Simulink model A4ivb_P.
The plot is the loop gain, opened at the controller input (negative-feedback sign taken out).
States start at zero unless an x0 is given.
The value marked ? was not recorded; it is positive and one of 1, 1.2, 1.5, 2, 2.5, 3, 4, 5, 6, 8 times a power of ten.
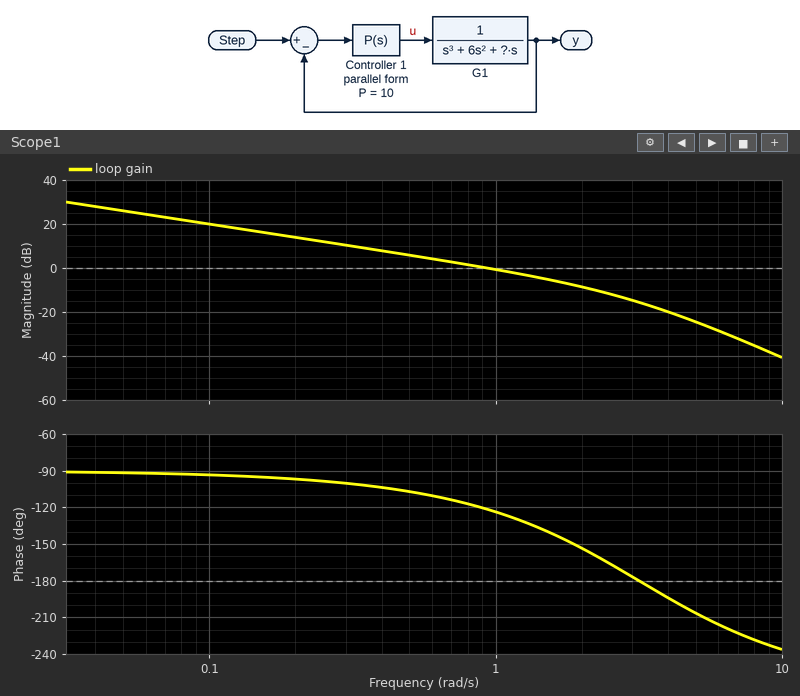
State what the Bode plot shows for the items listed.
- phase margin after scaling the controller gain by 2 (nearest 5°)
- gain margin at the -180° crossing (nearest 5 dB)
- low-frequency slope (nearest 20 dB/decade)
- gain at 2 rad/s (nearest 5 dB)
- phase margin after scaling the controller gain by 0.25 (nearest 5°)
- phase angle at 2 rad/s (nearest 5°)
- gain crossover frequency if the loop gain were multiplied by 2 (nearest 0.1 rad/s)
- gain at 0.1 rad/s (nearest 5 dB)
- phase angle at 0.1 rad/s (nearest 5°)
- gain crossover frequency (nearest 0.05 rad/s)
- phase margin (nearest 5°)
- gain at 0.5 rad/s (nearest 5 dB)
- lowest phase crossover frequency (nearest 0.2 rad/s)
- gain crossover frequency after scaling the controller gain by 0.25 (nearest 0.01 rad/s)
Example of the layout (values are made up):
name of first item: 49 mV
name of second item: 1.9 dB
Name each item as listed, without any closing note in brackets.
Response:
phase margin after scaling the controller gain by 2: 35°
gain margin at the -180° crossing: 15 dB
low-frequency slope: -20 dB/decade
gain at 2 rad/s: -10 dB
phase margin after scaling the controller gain by 0.25: 80°
phase angle at 2 rad/s: -155°
gain crossover frequency if the loop gain were multiplied by 2: 1.6 rad/s
gain at 0.1 rad/s: 20 dB
phase angle at 0.1 rad/s: -95°
gain crossover frequency: 0.95 rad/s
phase margin: 60°
gain at 0.5 rad/s: 5 dB
lowest phase crossover frequency: 3.2 rad/s
gain crossover frequency after scaling the controller gain by 0.25: 0.25 rad/s
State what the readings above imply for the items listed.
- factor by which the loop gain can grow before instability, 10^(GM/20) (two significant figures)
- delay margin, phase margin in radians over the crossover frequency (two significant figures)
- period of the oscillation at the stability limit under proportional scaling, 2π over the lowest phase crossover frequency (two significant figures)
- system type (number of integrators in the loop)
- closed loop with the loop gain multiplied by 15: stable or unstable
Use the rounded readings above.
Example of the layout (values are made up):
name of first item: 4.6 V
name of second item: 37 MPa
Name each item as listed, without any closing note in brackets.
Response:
factor by which the loop gain can grow before instability, 10^(GM/20): 5.6
delay margin, phase margin in radians over the crossover frequency: 1.1 s
period of the oscillation at the stability limit under proportional scaling, 2π over the lowest phase crossover frequency: 2.0 s
system type: 1
closed loop with the loop gain multiplied by 15: stable or unstable: unstable
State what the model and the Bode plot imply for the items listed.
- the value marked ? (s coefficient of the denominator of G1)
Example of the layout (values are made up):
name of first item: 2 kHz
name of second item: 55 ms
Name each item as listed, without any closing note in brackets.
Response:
the value marked ?: 10
